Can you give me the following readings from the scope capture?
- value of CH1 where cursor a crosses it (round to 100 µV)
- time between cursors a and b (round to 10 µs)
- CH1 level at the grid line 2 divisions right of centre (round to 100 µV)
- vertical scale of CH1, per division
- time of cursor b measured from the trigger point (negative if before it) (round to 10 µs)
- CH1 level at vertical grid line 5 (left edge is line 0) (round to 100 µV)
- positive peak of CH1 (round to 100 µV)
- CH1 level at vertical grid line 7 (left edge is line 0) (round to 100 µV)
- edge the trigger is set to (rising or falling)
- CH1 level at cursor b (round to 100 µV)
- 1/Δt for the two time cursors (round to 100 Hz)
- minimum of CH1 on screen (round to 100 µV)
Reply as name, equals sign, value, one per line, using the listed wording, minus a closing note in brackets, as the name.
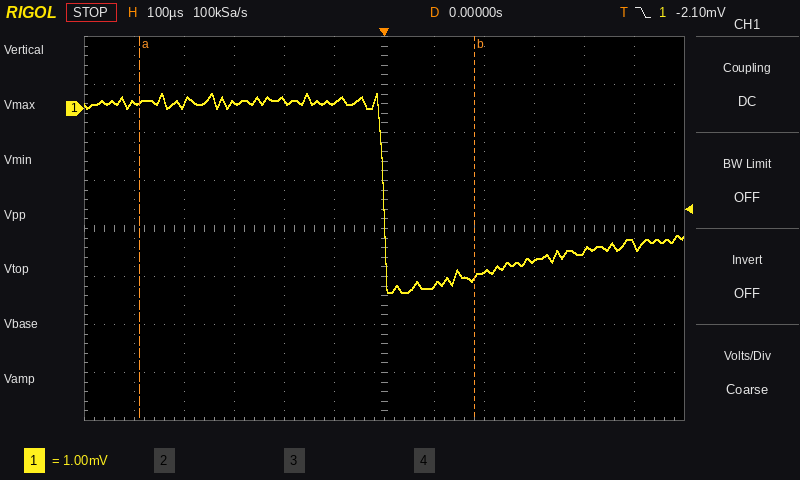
value of CH1 where cursor a crosses it = 100 µV
time between cursors a and b = 670 µs
CH1 level at the grid line 2 divisions right of centre = -3.4 mV
vertical scale of CH1, per division = 1 mV
time of cursor b measured from the trigger point (negative if before it) = +180 µs
CH1 level at vertical grid line 5 (left edge is line 0) = 100 µV
positive peak of CH1 = 300 µV
CH1 level at vertical grid line 7 (left edge is line 0) = -3.7 mV
edge the trigger is set to = falling
CH1 level at cursor b = -3.5 mV
1/Δt for the two time cursors = 1.5 kHz
minimum of CH1 on screen = -3.8 mV
